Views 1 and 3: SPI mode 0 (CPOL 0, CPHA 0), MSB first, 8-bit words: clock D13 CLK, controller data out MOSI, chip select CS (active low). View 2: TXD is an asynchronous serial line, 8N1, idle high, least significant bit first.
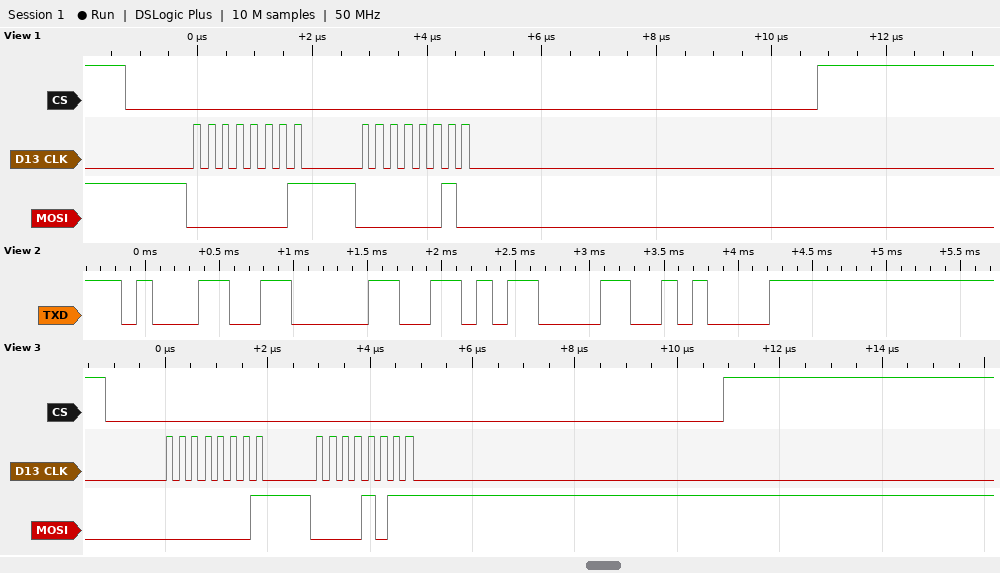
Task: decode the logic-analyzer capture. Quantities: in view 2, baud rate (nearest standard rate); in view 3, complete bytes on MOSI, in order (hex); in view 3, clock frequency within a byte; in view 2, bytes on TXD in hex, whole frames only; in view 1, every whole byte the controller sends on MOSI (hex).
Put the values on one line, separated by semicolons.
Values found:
9600 baud; 01 0B; 4 MHz; 0x31 0x30 0x0D 0x0A; 0x01 0x02
